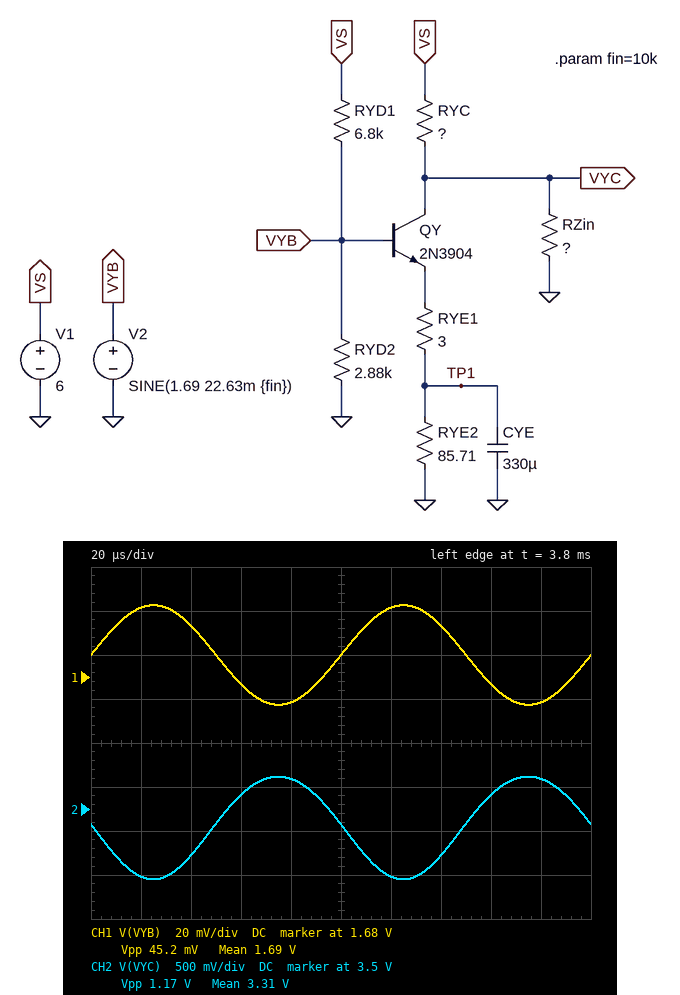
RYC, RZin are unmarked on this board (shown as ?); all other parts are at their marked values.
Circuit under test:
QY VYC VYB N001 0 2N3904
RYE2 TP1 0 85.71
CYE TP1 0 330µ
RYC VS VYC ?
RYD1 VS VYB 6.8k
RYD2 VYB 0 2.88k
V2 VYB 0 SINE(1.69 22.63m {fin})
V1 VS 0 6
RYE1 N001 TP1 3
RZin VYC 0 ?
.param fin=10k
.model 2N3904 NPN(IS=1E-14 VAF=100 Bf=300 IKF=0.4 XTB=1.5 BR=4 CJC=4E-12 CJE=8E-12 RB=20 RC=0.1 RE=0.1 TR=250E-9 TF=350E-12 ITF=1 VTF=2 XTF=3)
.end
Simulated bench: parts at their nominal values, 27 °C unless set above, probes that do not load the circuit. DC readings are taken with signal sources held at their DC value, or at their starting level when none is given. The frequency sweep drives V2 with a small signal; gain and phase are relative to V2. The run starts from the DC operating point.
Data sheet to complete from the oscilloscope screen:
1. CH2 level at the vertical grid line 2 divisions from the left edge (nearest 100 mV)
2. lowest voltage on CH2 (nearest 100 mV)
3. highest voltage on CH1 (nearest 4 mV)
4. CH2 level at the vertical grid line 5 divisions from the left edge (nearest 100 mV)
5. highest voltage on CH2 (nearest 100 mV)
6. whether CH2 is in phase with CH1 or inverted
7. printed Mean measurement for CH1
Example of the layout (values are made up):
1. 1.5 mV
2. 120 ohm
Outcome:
1. 3.0 V
2. 2.7 V
3. 1.712 V
4. 3.3 V
5. 3.9 V
6. inverted
7. 1.69 V
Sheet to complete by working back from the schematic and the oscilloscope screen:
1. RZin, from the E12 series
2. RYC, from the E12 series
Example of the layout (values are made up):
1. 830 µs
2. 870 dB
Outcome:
1. 820 Ω
2. 180 Ω
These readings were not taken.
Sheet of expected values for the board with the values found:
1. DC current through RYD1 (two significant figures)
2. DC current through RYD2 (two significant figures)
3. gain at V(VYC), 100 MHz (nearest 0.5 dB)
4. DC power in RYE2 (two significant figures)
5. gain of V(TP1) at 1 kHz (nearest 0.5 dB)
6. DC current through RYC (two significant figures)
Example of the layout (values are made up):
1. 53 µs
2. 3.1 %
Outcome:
1. 630 µA
2. 590 µA
3. 21.0 dB
4. 10 mW
5. -21.5 dB
6. 15 mA
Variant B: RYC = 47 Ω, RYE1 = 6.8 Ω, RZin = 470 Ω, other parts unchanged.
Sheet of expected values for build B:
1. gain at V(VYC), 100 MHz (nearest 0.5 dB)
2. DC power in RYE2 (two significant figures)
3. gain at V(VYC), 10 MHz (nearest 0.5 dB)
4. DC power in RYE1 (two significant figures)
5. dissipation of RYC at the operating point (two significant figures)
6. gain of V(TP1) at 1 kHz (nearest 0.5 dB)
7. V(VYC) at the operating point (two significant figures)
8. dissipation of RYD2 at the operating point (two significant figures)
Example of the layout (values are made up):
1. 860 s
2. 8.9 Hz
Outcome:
1. 10.5 dB
2. 9.5 mW
3. 13.0 dB
4. 750 µW
5. 21 mW
6. -26.0 dB
7. 5.0 V
8. 990 µW
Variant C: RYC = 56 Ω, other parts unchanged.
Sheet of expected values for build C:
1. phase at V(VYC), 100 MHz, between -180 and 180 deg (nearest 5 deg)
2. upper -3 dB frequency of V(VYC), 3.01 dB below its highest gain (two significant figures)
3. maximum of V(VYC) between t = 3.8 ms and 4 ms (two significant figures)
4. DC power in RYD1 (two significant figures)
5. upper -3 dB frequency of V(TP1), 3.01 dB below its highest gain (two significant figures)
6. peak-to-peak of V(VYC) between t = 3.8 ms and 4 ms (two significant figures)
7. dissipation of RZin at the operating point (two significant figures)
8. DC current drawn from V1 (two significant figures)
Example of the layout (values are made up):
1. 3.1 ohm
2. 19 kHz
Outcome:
1. 125 deg
2. 77 MHz
3. 5.2 V
4. 2.7 mW
5. 92 Hz
6. 420 mV
7. 31 mW
8. 18 mA
